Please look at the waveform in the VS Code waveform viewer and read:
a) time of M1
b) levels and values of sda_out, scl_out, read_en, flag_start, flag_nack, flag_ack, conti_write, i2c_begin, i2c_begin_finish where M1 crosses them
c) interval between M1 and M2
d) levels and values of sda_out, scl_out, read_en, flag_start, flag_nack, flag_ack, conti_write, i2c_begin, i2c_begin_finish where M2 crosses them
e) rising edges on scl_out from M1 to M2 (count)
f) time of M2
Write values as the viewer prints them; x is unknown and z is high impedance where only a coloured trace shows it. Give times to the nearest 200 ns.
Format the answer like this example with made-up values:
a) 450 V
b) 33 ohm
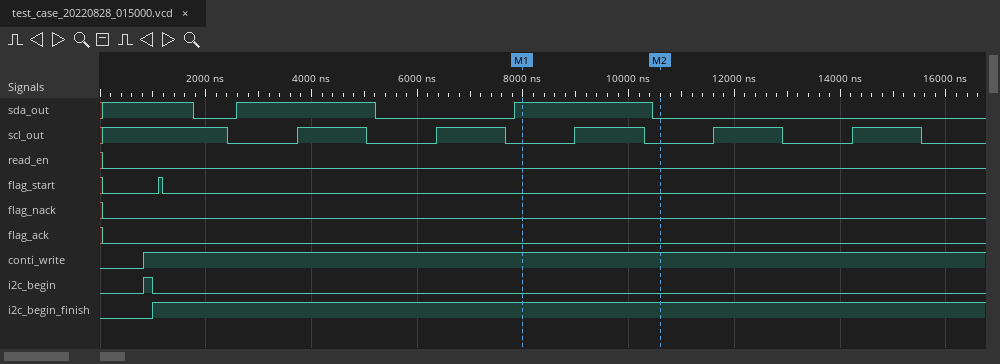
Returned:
a) 8000 ns
b) sda_out=1, scl_out=0, read_en=0, flag_start=0, flag_nack=0, flag_ack=0, conti_write=1, i2c_begin=0, i2c_begin_finish=1
c) 2600 ns
d) sda_out=0, scl_out=0, read_en=0, flag_start=0, flag_nack=0, flag_ack=0, conti_write=1, i2c_begin=0, i2c_begin_finish=1
e) 1
f) 10600 ns
